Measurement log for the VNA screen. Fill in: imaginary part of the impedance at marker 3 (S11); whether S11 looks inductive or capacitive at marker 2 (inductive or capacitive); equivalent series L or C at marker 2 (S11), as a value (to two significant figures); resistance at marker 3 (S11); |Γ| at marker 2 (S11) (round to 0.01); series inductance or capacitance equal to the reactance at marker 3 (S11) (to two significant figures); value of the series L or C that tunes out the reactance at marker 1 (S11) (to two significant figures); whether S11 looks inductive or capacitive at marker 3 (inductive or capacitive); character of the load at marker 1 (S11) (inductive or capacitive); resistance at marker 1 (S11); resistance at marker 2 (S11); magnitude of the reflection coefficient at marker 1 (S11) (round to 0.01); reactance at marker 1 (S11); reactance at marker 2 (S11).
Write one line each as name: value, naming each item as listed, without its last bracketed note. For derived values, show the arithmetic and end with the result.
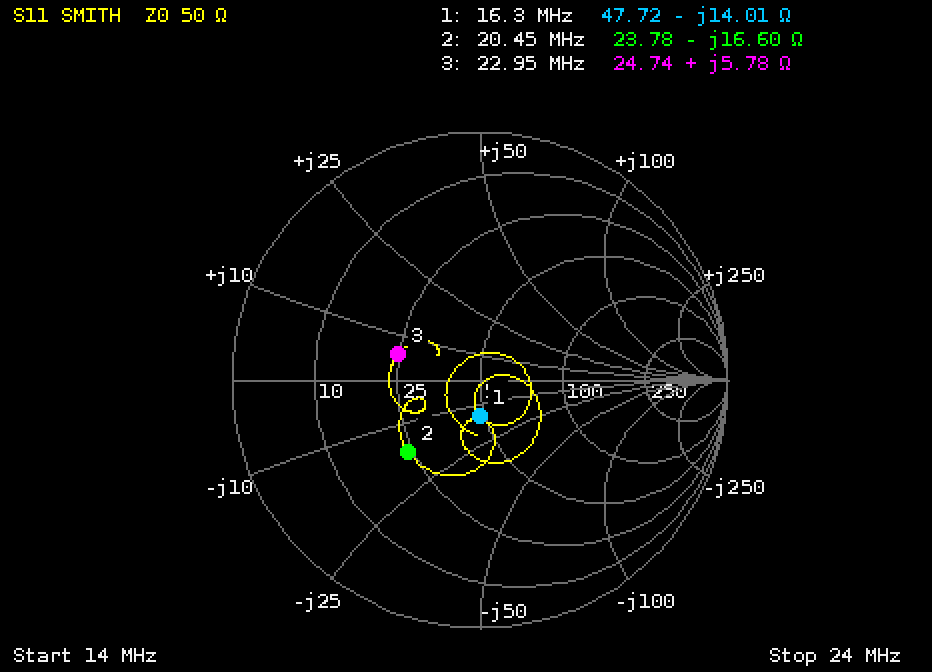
imaginary part of the impedance at marker 3: +5.78 Ω
whether S11 looks inductive or capacitive at marker 2: capacitive
equivalent series L or C at marker 2 (S11), as a value: C = 1/(2π × 20.45 MHz × 16.6 Ω) ≈ 469 pF, so 470 pF to two significant figures
resistance at marker 3: 24.74 Ω
|Γ| at marker 2 (S11): 0.41
series inductance or capacitance equal to the reactance at marker 3 (S11): L = 5.78 Ω/(2π × 22.95 MHz) ≈ 40 nH
value of the series L or C that tunes out the reactance at marker 1 (S11): L = 14.01 Ω/(2π × 16.3 MHz) ≈ 137 nH, so 140 nH to two significant figures
whether S11 looks inductive or capacitive at marker 3: inductive
character of the load at marker 1 (S11): capacitive
resistance at marker 1: 47.72 Ω
resistance at marker 2: 23.78 Ω
magnitude of the reflection coefficient at marker 1 (S11): 0.14
reactance at marker 1: -14.01 Ω
reactance at marker 2: -16.60 Ω
